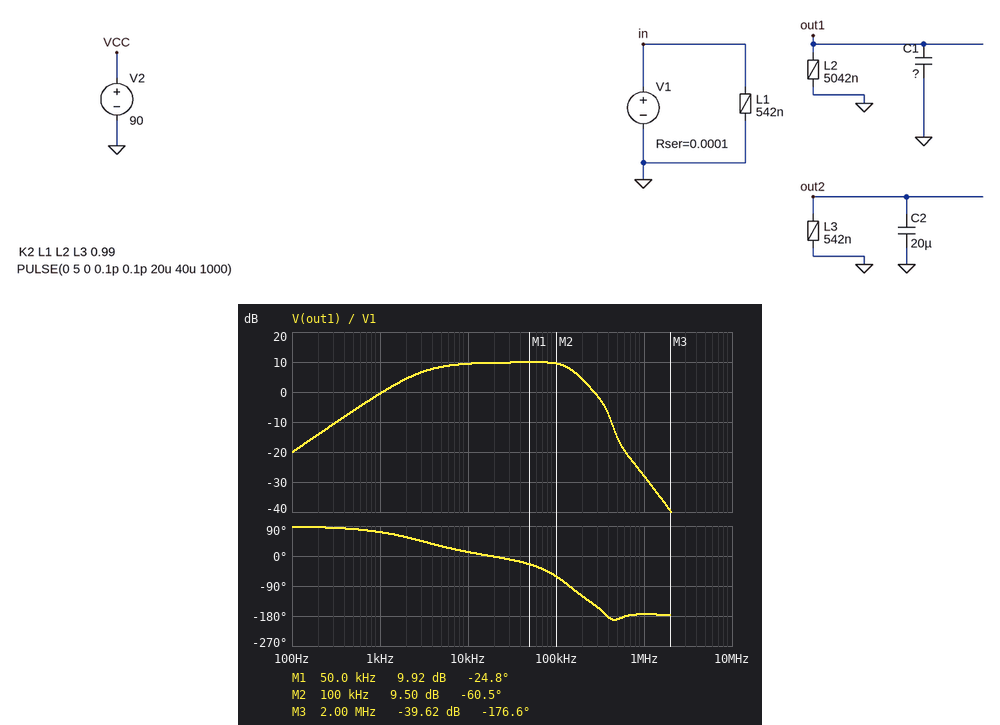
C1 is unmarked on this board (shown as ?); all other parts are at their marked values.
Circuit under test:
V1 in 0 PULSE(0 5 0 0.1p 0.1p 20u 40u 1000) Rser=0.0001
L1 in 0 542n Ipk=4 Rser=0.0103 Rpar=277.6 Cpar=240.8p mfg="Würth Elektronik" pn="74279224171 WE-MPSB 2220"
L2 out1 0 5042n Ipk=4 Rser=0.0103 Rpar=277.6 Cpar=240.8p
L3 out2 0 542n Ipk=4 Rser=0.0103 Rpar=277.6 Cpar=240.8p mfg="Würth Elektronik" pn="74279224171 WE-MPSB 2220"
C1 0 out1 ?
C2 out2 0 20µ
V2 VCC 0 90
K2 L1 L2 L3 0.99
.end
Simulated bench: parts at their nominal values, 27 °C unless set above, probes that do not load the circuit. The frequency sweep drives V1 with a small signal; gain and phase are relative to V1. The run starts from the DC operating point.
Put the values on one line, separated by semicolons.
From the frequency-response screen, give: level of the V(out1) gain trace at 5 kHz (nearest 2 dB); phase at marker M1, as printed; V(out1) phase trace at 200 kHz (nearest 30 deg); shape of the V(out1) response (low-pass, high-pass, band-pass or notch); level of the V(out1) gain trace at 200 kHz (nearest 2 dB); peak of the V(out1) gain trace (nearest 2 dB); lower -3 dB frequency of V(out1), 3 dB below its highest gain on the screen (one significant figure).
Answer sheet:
8 dB; -24.8 deg; -120 deg; band-pass; 4 dB; 10 dB; 3 kHz
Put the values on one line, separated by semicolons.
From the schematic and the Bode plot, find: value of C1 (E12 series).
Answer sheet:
12 µF
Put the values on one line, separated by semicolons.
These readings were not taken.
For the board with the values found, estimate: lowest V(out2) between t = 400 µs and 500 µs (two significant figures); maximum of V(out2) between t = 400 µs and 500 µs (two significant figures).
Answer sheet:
-3.0 V; 3.0 V
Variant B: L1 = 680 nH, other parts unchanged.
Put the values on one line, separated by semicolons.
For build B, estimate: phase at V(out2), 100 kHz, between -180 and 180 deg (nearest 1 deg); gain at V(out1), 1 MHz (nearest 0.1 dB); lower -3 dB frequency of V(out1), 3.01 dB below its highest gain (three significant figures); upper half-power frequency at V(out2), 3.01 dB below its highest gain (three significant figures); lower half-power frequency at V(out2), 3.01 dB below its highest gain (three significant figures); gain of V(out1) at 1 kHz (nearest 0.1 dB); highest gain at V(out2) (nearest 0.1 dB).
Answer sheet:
-57 deg; -28.9 dB; 3.27 kHz; 126 kHz; 2.47 kHz; 0.2 dB; -0.9 dB
